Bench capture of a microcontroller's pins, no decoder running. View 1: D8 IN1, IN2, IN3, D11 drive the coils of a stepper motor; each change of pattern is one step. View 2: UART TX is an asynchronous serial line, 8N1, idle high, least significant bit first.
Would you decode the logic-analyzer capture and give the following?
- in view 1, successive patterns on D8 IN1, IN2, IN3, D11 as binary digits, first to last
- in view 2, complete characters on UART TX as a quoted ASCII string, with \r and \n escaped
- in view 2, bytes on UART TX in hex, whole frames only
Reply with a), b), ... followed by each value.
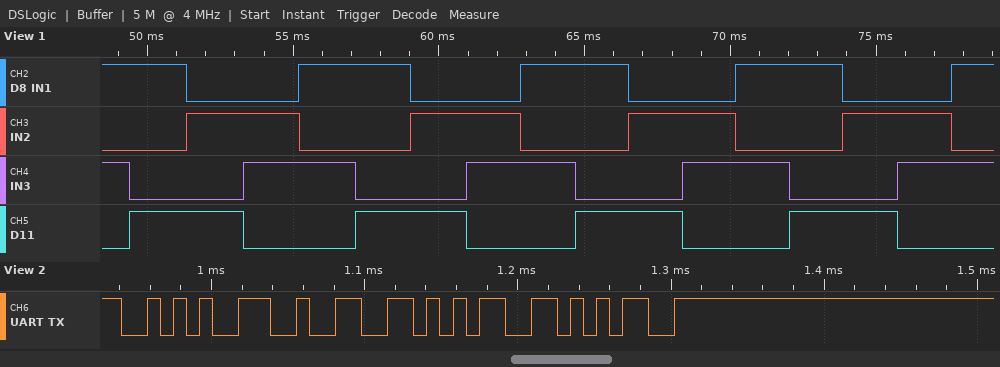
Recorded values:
a) 1010 1001 0101 0110 1010 1001 0101 0110 1010 1001 0101 0110 1010 1001 0101 0110 1010
b) "*255"
c) 2A 32 35 35
